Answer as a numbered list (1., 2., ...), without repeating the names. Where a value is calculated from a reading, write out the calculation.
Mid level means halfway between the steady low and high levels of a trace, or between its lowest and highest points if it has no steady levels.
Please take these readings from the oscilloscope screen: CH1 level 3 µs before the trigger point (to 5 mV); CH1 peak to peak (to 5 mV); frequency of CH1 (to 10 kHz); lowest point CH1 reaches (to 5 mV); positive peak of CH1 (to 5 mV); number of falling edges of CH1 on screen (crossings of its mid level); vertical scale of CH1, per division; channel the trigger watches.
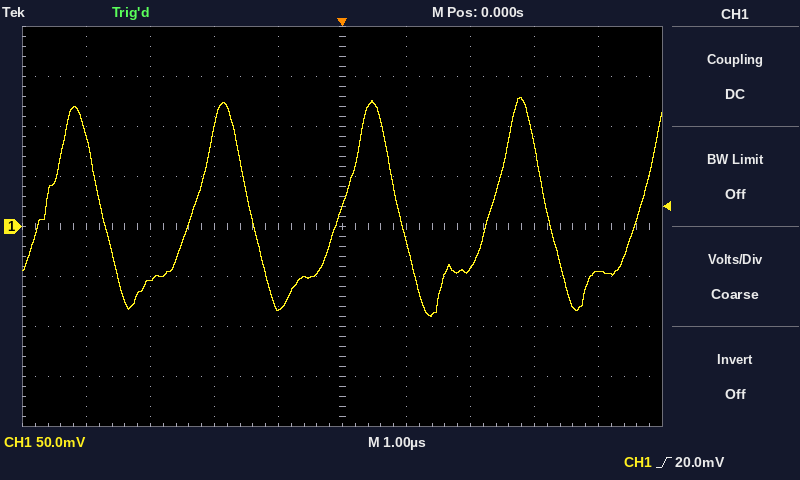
1. -55 mV
2. 130 mV − (-90 mV) = 220 mV
3. 430 kHz
4. -90 mV
5. 130 mV
6. 4
7. 50 mV
8. CH1
